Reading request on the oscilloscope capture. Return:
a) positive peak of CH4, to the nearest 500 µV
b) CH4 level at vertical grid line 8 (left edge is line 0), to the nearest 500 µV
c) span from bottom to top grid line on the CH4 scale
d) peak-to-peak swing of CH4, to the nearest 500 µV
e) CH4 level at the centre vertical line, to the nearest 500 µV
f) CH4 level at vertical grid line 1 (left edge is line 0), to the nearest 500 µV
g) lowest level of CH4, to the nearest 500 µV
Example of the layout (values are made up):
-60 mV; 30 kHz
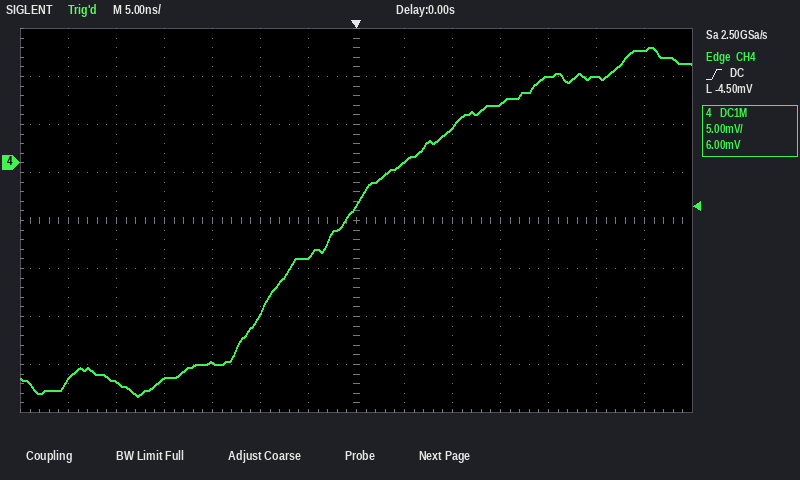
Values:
12.0 mV; 0.0 mV; 40 mV; 36.5 mV; -4.5 mV; -22.5 mV; -24.5 mV
